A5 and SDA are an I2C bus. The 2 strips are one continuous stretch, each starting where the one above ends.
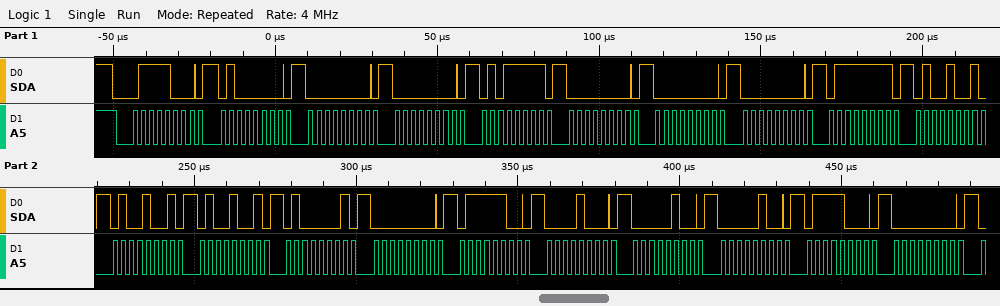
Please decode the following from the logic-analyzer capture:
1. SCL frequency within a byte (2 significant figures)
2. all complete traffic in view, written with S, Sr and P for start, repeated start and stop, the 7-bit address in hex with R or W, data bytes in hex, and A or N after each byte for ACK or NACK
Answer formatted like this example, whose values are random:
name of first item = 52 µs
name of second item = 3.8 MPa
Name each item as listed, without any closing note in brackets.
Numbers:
SCL frequency within a byte = 400 kHz
all complete traffic in view, written with S, Sr and P for start, repeated start and stop, the 7-bit address in hex with R or W, data bytes in hex, and A or N after each byte for ACK or NACK = S 3CW A 40 A 00 A 00 A 5F A 00 A 00 A 00 A 7F A 49 A 49 A 49 A 41 A 00 A 7C A 08 A 04 A 04 A 78 A 00 A
